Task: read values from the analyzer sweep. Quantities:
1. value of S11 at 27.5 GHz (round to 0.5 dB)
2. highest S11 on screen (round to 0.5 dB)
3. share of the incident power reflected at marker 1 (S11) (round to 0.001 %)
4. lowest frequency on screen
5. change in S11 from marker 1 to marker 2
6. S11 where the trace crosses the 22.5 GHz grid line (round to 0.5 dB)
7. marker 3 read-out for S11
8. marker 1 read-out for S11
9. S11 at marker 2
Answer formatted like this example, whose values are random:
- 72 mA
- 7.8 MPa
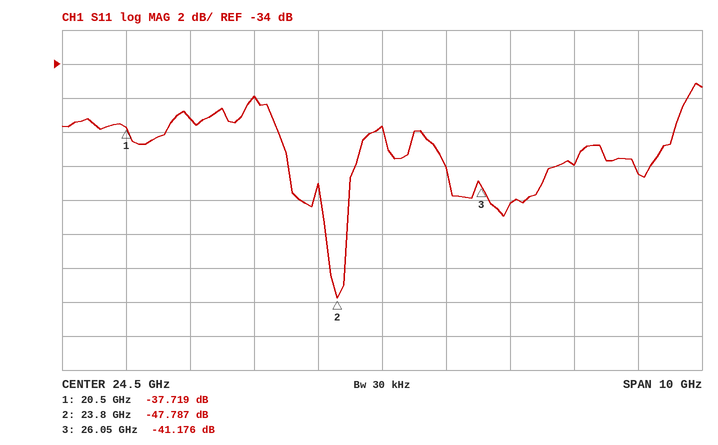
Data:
- -40.0 dB
- -35.0 dB
- 0.017 %
- 19.5 GHz
- -10.068 dB
- -36.0 dB
- -41.176 dB
- -37.719 dB
- -47.787 dB
